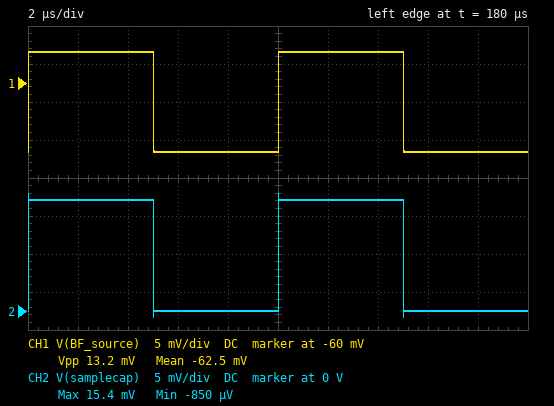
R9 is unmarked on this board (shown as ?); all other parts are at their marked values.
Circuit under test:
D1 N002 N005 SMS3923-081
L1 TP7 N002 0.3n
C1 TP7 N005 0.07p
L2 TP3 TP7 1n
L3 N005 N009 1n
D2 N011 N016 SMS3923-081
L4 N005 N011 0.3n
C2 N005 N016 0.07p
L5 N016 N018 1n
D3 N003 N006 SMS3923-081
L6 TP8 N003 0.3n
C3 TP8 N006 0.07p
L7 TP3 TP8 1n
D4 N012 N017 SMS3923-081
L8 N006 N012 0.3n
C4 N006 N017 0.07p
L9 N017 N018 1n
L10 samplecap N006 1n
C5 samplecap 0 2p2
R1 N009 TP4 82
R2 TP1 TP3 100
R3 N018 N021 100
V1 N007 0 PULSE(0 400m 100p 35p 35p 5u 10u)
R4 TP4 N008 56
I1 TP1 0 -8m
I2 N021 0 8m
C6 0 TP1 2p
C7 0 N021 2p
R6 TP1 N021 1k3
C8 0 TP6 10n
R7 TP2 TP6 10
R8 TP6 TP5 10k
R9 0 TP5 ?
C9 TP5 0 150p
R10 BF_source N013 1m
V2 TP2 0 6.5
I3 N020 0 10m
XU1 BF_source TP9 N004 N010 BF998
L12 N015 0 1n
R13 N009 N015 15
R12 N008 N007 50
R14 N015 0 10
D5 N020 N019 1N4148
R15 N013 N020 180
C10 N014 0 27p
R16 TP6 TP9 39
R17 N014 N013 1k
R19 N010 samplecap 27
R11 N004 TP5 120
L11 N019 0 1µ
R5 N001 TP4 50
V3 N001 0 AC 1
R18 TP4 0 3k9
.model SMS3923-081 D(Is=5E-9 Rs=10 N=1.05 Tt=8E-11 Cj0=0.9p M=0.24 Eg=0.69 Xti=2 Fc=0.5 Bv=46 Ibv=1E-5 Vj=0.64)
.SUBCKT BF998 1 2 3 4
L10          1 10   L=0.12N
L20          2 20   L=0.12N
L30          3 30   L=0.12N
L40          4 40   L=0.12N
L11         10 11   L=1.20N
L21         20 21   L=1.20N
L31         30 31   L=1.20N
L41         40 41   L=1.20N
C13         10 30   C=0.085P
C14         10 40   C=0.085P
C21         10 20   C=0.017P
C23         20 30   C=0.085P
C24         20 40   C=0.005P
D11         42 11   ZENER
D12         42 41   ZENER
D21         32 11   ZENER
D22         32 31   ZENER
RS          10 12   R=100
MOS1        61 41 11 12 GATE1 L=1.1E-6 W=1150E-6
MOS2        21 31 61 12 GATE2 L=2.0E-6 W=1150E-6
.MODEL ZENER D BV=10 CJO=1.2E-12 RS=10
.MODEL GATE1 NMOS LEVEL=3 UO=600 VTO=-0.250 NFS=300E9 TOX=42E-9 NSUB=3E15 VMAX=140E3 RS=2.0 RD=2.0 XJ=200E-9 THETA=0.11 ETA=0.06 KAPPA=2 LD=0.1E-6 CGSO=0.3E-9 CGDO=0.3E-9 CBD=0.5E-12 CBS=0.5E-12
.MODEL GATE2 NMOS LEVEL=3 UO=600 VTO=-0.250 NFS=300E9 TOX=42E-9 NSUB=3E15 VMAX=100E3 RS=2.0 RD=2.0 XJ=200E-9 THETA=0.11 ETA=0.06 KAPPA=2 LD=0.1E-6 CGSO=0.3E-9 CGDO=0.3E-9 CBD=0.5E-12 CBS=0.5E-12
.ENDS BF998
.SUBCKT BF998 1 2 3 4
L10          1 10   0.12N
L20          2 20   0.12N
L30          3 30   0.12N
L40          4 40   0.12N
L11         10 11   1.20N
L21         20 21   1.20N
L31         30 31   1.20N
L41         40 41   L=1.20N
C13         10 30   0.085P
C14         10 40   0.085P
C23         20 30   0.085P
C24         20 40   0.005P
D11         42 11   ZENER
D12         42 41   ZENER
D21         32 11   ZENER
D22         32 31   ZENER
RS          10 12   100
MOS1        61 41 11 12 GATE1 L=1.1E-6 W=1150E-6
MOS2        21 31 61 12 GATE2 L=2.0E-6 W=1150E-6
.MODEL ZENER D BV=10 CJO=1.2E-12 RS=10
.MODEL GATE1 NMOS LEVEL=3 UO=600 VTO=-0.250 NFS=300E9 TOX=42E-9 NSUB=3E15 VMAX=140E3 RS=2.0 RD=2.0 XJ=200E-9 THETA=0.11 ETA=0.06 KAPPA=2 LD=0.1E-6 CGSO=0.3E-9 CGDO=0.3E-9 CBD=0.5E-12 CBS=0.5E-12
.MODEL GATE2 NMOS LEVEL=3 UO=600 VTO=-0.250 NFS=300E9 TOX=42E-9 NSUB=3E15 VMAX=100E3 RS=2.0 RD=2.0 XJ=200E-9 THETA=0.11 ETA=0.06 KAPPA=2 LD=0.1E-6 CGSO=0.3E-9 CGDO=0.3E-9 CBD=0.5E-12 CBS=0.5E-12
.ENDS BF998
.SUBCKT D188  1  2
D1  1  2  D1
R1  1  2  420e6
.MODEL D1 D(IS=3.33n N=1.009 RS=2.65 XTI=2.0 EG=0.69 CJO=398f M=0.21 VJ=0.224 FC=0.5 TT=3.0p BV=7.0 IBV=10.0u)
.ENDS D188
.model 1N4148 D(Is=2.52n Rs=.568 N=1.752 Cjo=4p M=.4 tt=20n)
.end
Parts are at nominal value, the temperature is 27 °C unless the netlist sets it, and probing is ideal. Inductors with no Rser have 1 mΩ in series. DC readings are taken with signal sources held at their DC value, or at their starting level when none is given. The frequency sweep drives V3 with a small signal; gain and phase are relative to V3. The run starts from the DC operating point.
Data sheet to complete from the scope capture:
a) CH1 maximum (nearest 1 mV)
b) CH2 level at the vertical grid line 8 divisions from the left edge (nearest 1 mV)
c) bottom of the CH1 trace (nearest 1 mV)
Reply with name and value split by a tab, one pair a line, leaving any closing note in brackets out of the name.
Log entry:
CH1 maximum	-56 mV
CH2 level at the vertical grid line 8 divisions from the left edge	0 V
bottom of the CH1 trace	-69 mV
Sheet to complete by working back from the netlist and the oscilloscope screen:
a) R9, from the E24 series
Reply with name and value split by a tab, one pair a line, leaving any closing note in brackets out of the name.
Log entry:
R9, from the E24 series	13 kΩ
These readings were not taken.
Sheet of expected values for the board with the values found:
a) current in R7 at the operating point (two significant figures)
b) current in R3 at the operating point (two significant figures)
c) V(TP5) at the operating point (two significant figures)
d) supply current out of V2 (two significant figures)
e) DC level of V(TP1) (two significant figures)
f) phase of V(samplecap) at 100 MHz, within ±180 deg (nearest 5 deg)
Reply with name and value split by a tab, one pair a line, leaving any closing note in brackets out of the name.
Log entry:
current in R7 at the operating point	10 mA
current in R3 at the operating point	6.4 mA
V(TP5) at the operating point	3.6 V
supply current out of V2	10 mA
DC level of V(TP1)	1.0 V
phase of V(samplecap) at 100 MHz, within ±180 deg	-5 deg
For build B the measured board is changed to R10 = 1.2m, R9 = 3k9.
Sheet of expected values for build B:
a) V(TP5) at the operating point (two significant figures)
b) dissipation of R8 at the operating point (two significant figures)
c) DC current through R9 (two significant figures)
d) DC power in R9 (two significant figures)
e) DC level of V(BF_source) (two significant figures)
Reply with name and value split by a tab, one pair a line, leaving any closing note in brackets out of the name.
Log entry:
V(TP5) at the operating point	1.8 V
dissipation of R8 at the operating point	2.1 mW
DC current through R9	460 µA
DC power in R9	830 µW
DC level of V(BF_source)	-240 mV
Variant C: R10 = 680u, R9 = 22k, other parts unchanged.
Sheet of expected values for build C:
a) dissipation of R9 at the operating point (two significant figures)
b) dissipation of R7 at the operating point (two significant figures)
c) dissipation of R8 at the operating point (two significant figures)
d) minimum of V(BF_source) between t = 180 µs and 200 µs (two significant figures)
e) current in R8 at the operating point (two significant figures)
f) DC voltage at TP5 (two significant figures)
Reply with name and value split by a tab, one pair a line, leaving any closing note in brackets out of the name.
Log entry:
dissipation of R9 at the operating point	880 µW
dissipation of R7 at the operating point	1.0 mW
dissipation of R8 at the operating point	400 µW
minimum of V(BF_source) between t = 180 µs and 200 µs	3.3 mV
current in R8 at the operating point	200 µA
DC voltage at TP5	4.4 V
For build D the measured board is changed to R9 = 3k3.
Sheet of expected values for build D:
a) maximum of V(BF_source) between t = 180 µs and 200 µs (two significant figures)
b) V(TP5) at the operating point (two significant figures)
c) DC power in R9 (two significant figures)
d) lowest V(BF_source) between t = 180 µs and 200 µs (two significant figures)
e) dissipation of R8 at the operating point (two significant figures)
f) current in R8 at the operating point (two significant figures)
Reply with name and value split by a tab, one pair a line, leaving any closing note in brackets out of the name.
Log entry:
maximum of V(BF_source) between t = 180 µs and 200 µs	-240 mV
V(TP5) at the operating point	1.6 V
DC power in R9	760 µW
lowest V(BF_source) between t = 180 µs and 200 µs	-260 mV
dissipation of R8 at the operating point	2.3 mW
current in R8 at the operating point	480 µA
